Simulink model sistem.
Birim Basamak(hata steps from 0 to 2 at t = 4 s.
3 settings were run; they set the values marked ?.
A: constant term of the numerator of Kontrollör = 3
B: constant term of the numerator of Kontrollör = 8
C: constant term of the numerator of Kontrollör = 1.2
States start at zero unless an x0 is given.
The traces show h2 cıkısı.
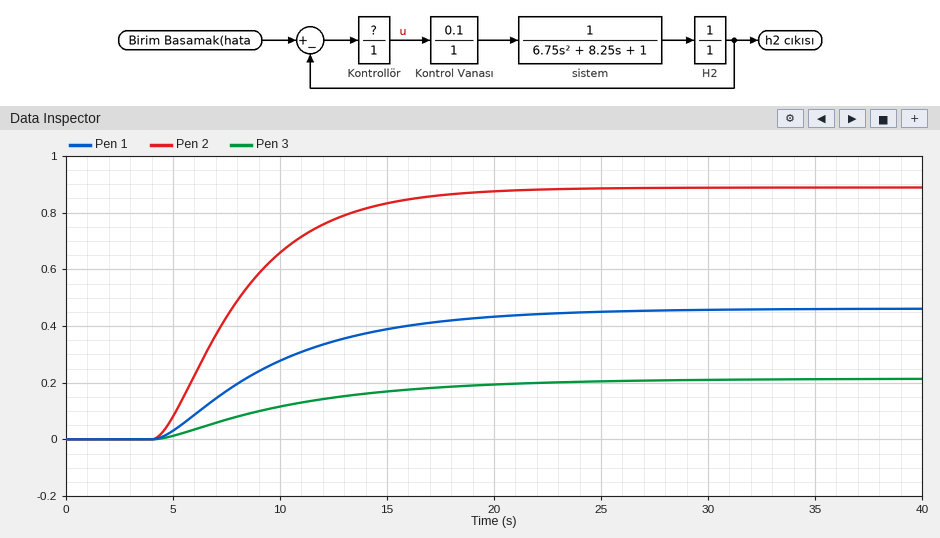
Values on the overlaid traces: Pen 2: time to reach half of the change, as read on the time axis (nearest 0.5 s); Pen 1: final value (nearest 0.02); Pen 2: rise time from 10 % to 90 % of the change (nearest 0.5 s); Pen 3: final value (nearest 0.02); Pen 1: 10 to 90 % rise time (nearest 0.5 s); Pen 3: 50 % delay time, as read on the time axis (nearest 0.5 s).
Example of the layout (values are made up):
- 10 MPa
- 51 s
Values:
- 7.5 s
- 0.46
- 8.5 s
- 0.22
- 12.0 s
- 9.5 s
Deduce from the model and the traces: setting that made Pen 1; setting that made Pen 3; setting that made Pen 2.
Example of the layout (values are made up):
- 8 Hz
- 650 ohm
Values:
- A
- C
- B
